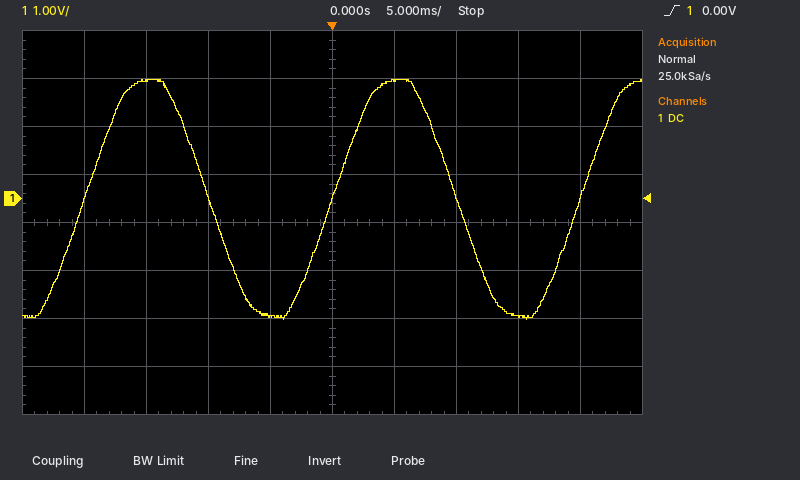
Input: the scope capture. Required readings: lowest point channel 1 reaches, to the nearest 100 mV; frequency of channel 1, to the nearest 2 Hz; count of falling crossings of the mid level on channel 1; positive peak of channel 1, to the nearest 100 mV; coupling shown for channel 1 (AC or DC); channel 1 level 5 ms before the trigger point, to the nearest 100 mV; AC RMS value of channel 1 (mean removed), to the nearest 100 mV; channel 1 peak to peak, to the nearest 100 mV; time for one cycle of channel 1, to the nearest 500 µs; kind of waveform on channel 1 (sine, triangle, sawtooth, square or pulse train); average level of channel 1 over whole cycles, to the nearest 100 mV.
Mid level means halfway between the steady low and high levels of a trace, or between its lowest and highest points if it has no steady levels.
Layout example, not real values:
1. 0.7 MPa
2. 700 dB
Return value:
1. -2.5 V
2. 50 Hz
3. 2
4. 2.5 V
5. DC
6. -2.4 V
7. 1.8 V
8. 5.0 V
9. 20.0 ms
10. sine
11. 0.0 V
